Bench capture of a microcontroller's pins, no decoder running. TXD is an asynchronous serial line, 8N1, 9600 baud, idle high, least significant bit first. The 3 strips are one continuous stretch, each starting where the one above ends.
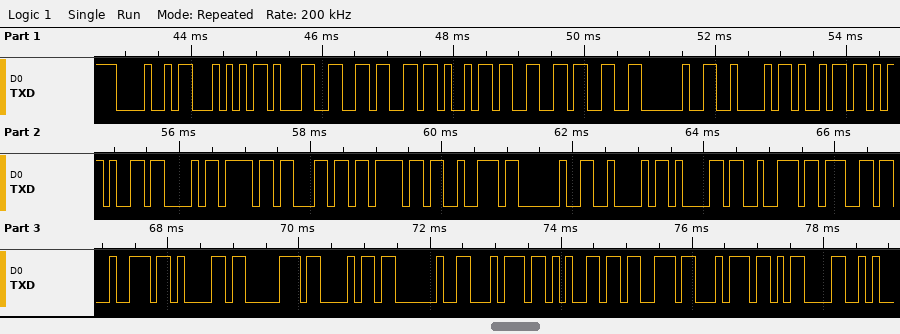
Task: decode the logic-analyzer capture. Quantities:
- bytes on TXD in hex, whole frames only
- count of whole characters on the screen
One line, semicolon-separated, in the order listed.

48 54 31 36 4B 33 33 20 42 69 2D 43 6F 6C 6F 72 20 42 61 72 67 72 61 70 68 20 74 65 73 74 0D; 31
